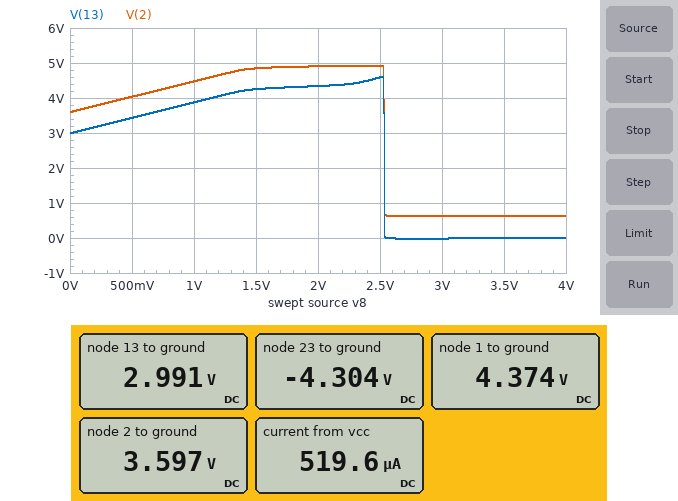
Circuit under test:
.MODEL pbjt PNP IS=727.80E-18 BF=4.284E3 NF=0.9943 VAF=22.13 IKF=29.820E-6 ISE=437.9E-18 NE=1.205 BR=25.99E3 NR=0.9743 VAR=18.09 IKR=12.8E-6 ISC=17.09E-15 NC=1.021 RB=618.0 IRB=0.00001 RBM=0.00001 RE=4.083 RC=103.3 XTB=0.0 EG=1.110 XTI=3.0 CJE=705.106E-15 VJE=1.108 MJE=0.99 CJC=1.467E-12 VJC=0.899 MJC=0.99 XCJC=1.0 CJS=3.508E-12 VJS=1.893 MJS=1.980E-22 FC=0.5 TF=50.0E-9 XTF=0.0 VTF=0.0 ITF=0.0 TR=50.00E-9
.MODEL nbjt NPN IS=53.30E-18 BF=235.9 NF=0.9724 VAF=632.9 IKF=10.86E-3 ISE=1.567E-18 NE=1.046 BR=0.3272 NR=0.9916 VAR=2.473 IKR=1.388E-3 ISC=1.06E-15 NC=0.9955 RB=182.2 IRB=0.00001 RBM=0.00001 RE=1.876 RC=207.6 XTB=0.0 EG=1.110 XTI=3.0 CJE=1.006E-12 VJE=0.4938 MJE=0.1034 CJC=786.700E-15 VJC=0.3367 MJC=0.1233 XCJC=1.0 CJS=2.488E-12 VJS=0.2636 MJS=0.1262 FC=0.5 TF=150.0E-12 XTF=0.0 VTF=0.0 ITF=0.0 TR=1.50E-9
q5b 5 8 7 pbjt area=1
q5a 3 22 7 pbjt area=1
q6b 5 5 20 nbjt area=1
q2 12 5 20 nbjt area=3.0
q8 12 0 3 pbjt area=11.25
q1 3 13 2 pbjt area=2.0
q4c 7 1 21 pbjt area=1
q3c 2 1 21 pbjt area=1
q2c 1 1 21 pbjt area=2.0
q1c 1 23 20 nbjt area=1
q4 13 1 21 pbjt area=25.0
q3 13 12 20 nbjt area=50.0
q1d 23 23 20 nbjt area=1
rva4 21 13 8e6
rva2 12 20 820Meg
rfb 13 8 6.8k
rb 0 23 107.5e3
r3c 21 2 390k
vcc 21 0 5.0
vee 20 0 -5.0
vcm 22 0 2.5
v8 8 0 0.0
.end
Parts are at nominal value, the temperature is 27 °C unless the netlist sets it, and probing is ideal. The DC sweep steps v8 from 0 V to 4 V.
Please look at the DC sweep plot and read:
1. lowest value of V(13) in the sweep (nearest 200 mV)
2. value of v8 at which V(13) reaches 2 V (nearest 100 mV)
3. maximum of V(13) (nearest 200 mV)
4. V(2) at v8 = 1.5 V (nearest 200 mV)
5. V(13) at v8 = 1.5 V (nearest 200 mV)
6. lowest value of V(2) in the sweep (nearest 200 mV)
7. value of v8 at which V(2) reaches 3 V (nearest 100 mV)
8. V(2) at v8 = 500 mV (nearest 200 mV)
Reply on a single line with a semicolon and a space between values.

0 V; 2.5 V; 4.6 V; 4.8 V; 4.2 V; 600 mV; 2.5 V; 4.0 V
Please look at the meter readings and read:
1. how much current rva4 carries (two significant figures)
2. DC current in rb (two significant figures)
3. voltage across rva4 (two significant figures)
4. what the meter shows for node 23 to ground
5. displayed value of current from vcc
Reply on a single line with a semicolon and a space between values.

250 nA; 40 µA; 2.0 V; -4.304 V; 519.6 µA
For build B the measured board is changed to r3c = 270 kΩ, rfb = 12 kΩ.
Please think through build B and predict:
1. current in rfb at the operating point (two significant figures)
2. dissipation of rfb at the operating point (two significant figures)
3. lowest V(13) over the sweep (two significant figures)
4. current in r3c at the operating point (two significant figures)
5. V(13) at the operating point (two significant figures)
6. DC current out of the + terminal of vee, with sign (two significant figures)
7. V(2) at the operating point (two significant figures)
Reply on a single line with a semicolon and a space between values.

360 µA; 1.6 mW; -26 mV; 380 nA; 4.3 V; -100 µA; 4.9 V
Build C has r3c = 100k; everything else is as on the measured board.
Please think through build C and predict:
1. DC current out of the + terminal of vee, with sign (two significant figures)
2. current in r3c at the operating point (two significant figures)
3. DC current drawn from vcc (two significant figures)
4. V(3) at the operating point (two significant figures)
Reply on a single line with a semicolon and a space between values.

-130 µA; 14 µA; 530 µA; 560 mV
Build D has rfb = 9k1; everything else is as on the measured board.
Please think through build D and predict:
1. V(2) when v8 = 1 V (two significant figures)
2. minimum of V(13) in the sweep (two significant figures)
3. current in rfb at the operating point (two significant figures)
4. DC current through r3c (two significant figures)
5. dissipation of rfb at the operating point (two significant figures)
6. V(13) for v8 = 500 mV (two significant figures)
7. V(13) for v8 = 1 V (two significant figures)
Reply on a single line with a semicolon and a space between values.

4.9 V; -20 mV; 420 µA; 1.4 µA; 1.6 mW; 4.2 V; 4.3 V
